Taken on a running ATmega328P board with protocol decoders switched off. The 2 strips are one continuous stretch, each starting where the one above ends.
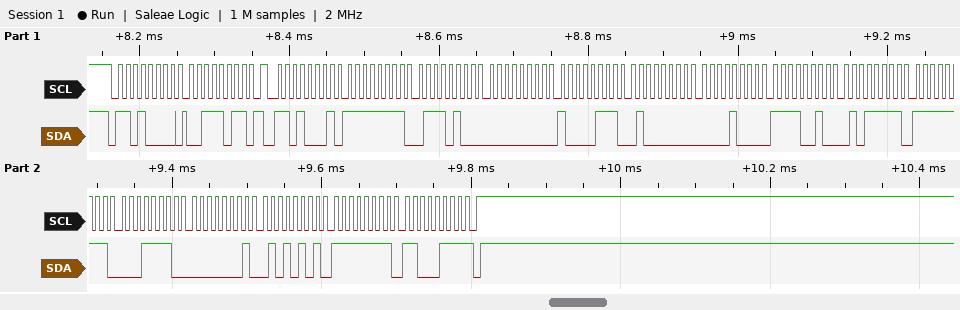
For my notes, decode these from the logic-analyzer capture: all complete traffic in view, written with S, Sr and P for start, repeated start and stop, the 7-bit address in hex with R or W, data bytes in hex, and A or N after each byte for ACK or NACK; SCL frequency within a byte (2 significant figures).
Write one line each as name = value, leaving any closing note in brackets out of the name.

all complete traffic in view, written with S, Sr and P for start, repeated start and stop, the 7-bit address in hex with R or W, data bytes in hex, and A or N after each byte for ACK or NACK = S 68W A 3B A Sr 68R A FF A 74 A 00 A 87 A 40 A 08 A F2 A 5F A FF A 1E A 01 A 55 A FF A C7 N P
SCL frequency within a byte = 100 kHz
